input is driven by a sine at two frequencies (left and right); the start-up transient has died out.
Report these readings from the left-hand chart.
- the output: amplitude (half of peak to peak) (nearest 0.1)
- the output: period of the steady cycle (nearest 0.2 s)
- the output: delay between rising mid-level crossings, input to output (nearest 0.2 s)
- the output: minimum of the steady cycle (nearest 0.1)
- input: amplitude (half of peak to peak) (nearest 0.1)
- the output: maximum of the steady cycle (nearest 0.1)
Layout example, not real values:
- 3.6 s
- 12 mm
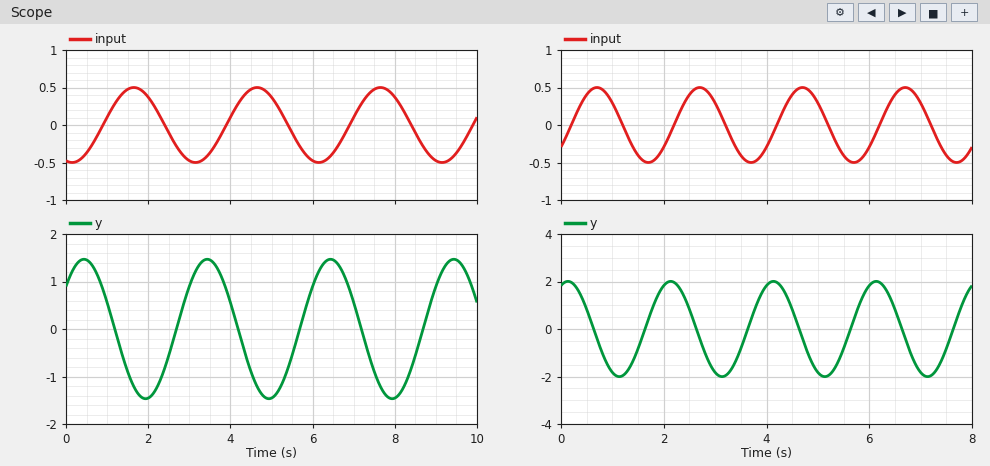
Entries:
- 1.5
- 3.0 s
- 1.8 s
- -1.5
- 0.5
- 1.5
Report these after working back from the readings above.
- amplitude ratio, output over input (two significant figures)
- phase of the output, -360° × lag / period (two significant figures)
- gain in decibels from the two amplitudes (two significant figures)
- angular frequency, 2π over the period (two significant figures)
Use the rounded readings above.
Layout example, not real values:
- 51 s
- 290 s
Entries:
- 3.0
- -220°
- 9.5 dB
- 2.1 rad/s
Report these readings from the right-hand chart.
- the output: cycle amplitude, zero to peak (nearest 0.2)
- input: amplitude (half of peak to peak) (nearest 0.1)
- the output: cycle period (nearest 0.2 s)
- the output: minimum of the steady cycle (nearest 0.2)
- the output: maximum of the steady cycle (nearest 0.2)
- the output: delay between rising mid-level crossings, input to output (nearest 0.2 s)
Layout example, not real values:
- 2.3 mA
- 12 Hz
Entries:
- 2.0
- 0.5
- 2.0 s
- -2.0
- 2.0
- 1.4 s
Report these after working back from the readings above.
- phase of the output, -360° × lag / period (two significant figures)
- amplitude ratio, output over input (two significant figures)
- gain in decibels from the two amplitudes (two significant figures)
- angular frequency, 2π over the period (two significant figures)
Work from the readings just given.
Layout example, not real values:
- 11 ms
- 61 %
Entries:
- -250°
- 4.0
- 12 dB
- 3.1 rad/s
